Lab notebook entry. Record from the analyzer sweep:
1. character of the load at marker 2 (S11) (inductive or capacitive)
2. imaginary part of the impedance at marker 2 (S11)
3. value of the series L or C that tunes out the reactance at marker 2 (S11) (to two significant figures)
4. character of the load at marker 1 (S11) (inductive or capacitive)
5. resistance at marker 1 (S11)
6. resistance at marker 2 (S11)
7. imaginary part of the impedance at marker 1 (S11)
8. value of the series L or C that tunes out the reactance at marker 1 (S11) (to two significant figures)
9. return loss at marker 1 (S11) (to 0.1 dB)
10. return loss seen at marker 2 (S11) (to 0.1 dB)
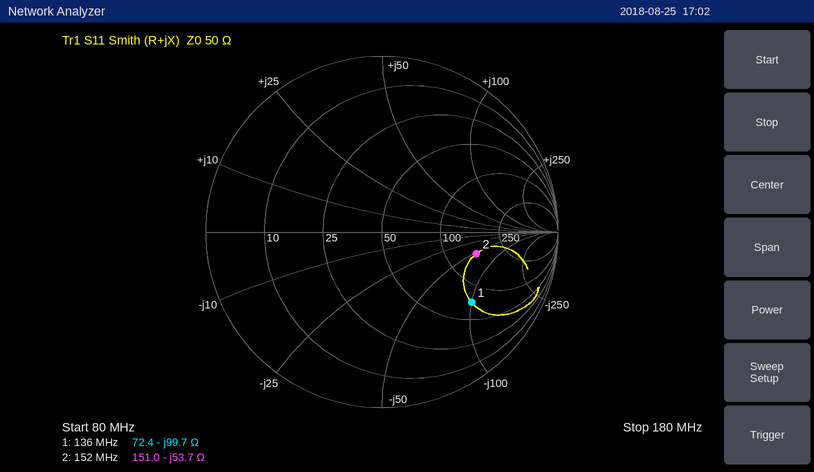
capacitive
-53.7 Ω
56 nH
capacitive
72.4 Ω
151.0 Ω
-99.7 Ω
120 nH
3.8 dB
5.2 dB
